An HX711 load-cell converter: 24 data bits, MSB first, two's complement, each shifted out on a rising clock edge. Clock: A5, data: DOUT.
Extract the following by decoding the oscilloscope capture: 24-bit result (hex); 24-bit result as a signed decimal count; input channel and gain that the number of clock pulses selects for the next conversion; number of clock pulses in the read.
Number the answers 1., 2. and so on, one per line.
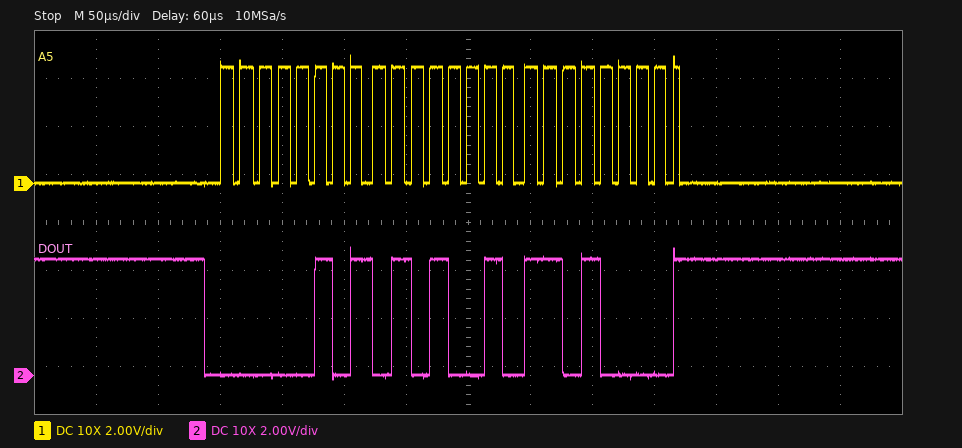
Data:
1. 0x0552D0
2. 348880
3. channel A, gain 128
4. 25
